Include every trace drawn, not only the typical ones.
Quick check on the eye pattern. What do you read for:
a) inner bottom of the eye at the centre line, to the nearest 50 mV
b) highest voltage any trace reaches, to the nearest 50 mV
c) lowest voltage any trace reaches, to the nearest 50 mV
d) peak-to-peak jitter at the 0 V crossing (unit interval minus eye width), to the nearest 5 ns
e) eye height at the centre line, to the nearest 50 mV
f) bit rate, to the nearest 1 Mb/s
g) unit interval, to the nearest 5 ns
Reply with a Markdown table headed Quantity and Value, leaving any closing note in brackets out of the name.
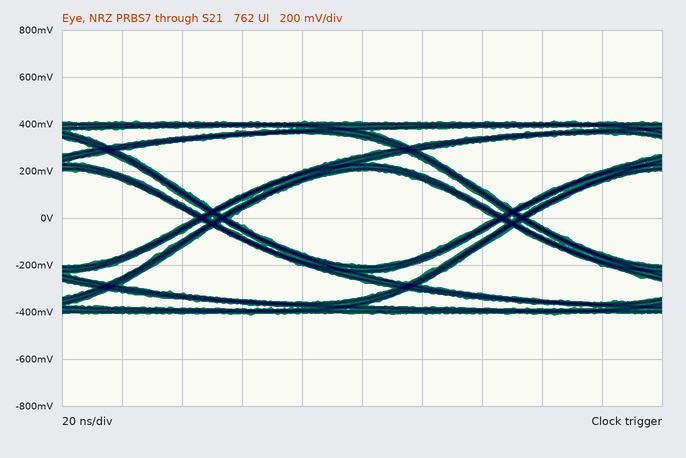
| Quantity | Value |
|---|---|
| inner bottom of the eye at the centre line, to the nearest 50 mV | -200 mV |
| highest voltage any trace reaches, to the nearest 50 mV | 400 mV |
| lowest voltage any trace reaches, to the nearest 50 mV | -400 mV |
| peak-to-peak jitter at the 0 V crossing (unit interval minus eye width), to the nearest 5 ns | 10 ns |
| eye height at the centre line, to the nearest 50 mV | 400 mV |
| bit rate, to the nearest 1 Mb/s | 10 Mb/s |
| unit interval, to the nearest 5 ns | 100 ns |
